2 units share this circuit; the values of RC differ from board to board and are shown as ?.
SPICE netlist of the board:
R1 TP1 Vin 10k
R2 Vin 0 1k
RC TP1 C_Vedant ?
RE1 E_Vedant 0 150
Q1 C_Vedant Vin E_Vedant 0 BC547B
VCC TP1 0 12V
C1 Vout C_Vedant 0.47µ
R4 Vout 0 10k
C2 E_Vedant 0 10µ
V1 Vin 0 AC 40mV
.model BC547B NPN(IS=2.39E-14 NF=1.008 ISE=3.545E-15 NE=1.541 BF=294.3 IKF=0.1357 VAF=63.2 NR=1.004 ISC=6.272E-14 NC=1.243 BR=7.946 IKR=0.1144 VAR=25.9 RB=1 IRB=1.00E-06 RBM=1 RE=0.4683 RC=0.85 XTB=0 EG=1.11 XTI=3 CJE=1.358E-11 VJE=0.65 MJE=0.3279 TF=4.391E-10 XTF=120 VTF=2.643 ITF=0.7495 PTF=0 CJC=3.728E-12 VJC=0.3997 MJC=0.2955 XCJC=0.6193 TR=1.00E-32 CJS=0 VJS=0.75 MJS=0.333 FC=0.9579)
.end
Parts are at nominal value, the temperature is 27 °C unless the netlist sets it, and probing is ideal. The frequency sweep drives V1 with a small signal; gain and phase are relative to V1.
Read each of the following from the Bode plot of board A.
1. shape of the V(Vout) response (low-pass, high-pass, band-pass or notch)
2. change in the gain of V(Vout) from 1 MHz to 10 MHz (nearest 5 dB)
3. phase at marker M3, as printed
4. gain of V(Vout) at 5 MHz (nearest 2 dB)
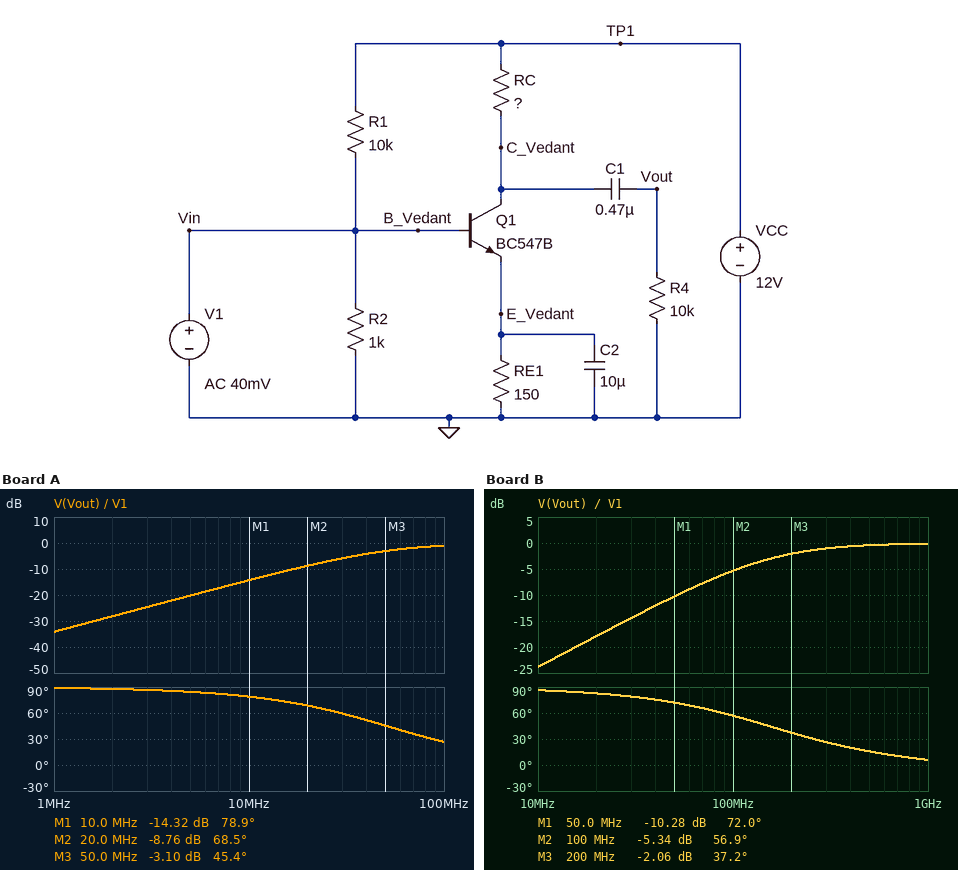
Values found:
high-pass
20 dB
45.4 deg
-20 dB
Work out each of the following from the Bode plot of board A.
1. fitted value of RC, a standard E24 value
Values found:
3 kΩ
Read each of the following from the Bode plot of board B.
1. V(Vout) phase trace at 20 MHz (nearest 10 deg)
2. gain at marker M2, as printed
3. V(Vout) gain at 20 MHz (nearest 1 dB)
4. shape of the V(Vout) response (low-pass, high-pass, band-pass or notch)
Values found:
80 deg
-5.34 dB
-18 dB
high-pass
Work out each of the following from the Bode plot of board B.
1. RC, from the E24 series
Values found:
820 Ω
